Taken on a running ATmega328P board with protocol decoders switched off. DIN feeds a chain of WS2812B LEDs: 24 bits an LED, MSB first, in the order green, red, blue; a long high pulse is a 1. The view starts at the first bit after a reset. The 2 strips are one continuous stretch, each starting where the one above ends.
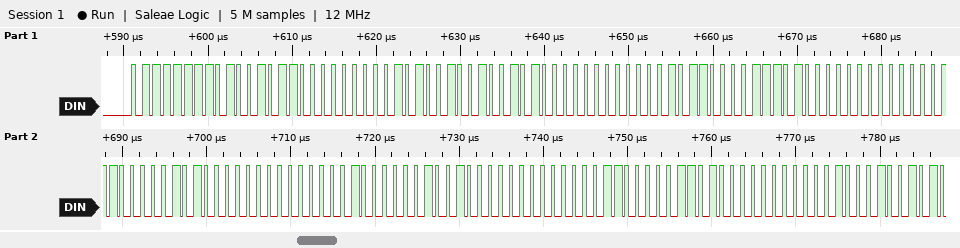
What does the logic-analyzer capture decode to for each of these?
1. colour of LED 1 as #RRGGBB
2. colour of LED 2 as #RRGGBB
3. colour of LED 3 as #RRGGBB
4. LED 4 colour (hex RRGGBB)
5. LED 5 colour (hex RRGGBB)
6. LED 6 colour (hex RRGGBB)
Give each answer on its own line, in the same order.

#4B7F00
#4A5200
#1D1600
#0A0600
#090400
#0D0600
